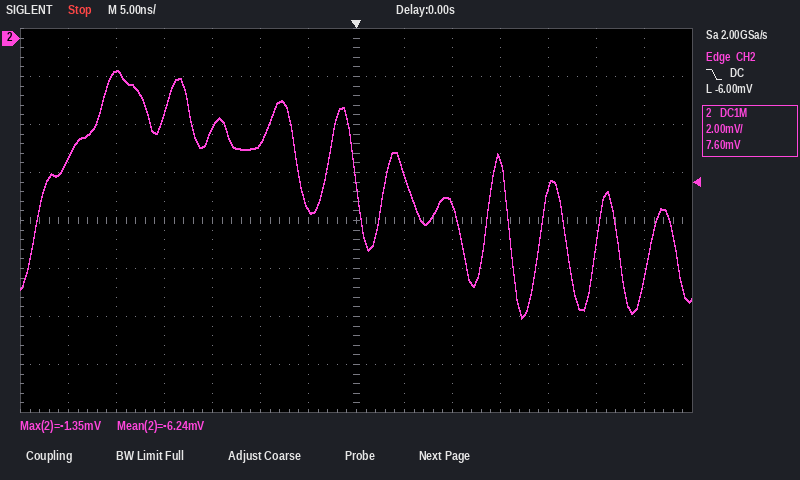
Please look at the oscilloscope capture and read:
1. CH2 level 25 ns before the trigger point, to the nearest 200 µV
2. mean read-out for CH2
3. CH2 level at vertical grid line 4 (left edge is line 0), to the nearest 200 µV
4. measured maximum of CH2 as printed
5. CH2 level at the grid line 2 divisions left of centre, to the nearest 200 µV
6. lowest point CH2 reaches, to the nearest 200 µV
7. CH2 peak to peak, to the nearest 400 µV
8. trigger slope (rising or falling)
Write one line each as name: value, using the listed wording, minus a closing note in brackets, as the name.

CH2 level 25 ns before the trigger point, to the nearest 200 µV: -1.4 mV
mean read-out for CH2: -6.24 mV
CH2 level at vertical grid line 4 (left edge is line 0), to the nearest 200 µV: -3.8 mV
measured maximum of CH2 as printed: -1.35 mV
CH2 level at the grid line 2 divisions left of centre, to the nearest 200 µV: -4.4 mV
lowest point CH2 reaches, to the nearest 200 µV: -11.6 mV
CH2 peak to peak, to the nearest 400 µV: 10.4 mV
trigger slope: falling
